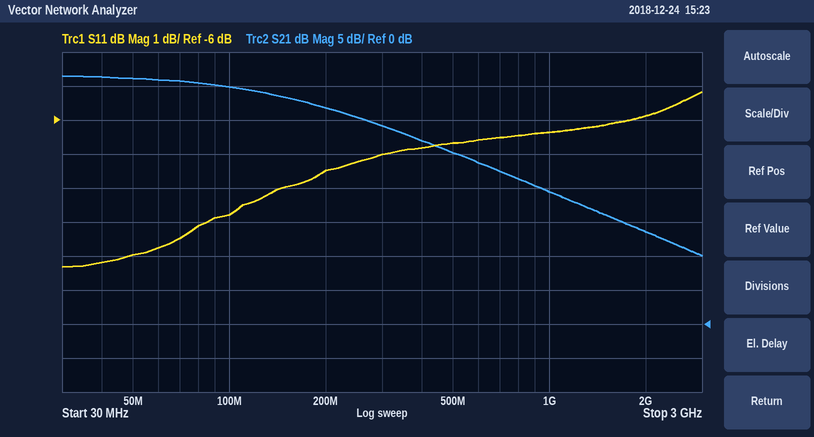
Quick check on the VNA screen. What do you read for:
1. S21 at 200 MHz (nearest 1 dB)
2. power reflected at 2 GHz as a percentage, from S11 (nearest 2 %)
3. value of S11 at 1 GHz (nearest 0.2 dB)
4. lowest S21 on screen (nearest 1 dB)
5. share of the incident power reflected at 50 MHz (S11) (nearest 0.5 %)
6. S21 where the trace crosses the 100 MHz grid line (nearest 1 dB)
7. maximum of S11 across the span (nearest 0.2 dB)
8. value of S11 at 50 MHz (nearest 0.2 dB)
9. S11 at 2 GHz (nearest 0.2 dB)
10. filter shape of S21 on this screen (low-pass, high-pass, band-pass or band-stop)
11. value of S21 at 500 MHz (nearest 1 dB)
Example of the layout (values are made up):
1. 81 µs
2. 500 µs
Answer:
1. 32 dB
2. 26 %
3. -6.4 dB
4. 10 dB
5. 10.0 %
6. 35 dB
7. -5.2 dB
8. -10.0 dB
9. -5.8 dB
10. low-pass
11. 25 dB
